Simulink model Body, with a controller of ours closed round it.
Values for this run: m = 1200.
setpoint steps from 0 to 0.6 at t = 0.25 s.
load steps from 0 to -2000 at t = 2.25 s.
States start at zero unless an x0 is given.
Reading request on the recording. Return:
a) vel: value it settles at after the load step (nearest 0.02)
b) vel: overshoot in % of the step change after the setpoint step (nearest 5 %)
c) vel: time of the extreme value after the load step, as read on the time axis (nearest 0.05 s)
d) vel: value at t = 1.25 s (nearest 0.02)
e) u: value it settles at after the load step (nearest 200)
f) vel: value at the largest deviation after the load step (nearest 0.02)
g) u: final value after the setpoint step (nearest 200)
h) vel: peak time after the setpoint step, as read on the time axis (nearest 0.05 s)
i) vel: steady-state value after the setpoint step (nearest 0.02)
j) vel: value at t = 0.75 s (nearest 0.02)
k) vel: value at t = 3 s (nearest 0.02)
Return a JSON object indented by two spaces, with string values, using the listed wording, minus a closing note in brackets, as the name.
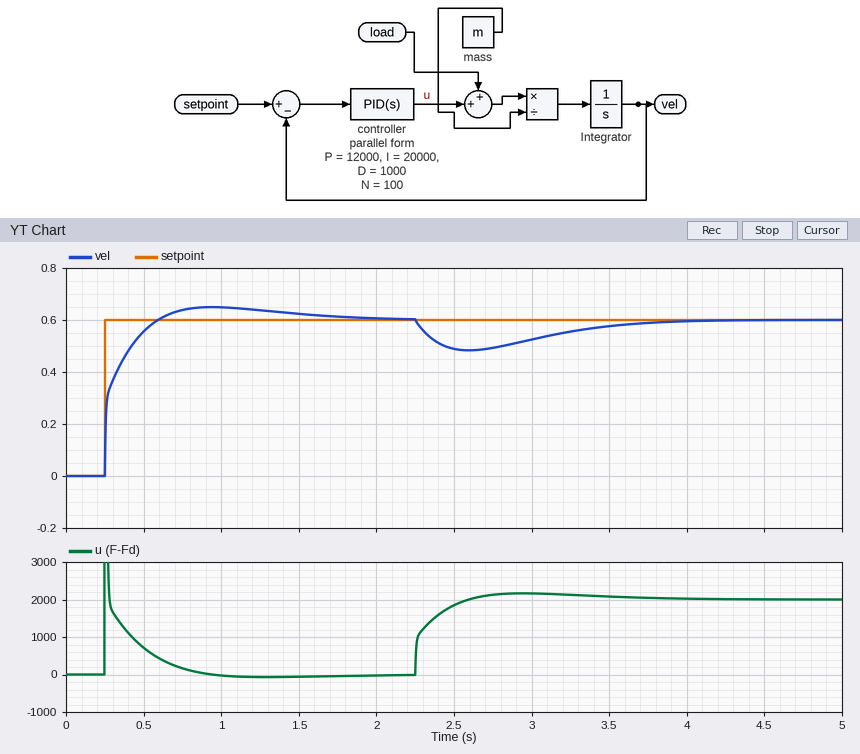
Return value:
{
  "vel: value it settles at after the load step": "0.60",
  "vel: overshoot in % of the step change after the setpoint step": "10 %",
  "vel: time of the extreme value after the load step, as read on the time axis": "2.60 s",
  "vel: value at t = 1.25 s": "0.64",
  "u: value it settles at after the load step": "2000",
  "vel: value at the largest deviation after the load step": "0.48",
  "u: final value after the setpoint step": "0",
  "vel: peak time after the setpoint step, as read on the time axis": "0.95 s",
  "vel: steady-state value after the setpoint step": "0.60",
  "vel: value at t = 0.75 s": "0.64",
  "vel: value at t = 3 s": "0.52"
}
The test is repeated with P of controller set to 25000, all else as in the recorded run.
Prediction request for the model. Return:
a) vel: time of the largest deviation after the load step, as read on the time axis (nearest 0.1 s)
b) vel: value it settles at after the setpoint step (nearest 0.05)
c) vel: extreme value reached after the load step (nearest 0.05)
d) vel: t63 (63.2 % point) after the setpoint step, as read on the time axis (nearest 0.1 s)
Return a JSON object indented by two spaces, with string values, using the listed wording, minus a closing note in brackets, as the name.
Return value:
{
  "vel: time of the largest deviation after the load step, as read on the time axis": "2.5 s",
  "vel: value it settles at after the setpoint step": "0.60",
  "vel: extreme value reached after the load step": "0.55",
  "vel: t63 (63.2 % point) after the setpoint step, as read on the time axis": "0.3 s"
}
